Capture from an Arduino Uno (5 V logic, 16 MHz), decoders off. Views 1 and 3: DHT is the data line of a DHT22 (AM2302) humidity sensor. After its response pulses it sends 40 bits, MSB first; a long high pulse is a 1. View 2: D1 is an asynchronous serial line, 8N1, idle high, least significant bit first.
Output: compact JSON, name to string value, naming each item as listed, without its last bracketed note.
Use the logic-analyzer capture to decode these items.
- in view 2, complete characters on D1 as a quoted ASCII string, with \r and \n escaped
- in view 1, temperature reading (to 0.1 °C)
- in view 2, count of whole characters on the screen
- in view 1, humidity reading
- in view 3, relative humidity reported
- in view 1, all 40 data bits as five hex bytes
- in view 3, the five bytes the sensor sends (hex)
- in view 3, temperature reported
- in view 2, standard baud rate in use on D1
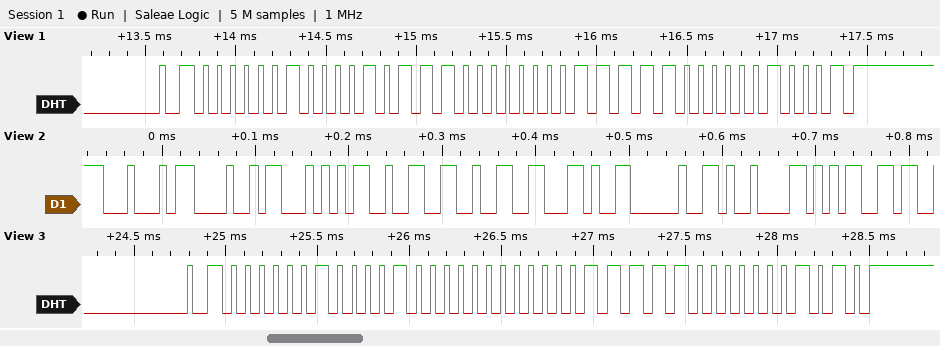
{"in view 2, complete characters on D1 as a quoted ASCII string, with \\r and \\n escaped": "\"DHT22, \\t5\"", "in view 1, temperature reading": "24.8 °C", "in view 2, count of whole characters on the screen": "9", "in view 1, humidity reading": "53.5 %", "in view 3, relative humidity reported": "52.8 %", "in view 1, all 40 data bits as five hex bytes": "02 17 00 F8 11", "in view 3, the five bytes the sensor sends": "02 10 00 F8 0A", "in view 3, temperature reported": "24.8 °C", "in view 2, standard baud rate in use on D1": "115200 baud"}
